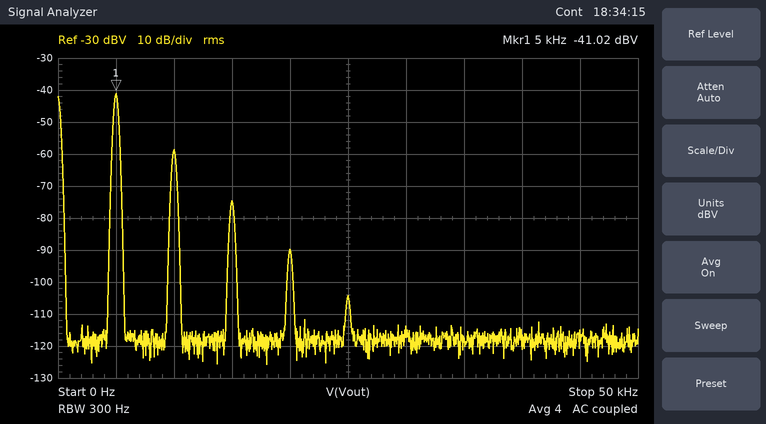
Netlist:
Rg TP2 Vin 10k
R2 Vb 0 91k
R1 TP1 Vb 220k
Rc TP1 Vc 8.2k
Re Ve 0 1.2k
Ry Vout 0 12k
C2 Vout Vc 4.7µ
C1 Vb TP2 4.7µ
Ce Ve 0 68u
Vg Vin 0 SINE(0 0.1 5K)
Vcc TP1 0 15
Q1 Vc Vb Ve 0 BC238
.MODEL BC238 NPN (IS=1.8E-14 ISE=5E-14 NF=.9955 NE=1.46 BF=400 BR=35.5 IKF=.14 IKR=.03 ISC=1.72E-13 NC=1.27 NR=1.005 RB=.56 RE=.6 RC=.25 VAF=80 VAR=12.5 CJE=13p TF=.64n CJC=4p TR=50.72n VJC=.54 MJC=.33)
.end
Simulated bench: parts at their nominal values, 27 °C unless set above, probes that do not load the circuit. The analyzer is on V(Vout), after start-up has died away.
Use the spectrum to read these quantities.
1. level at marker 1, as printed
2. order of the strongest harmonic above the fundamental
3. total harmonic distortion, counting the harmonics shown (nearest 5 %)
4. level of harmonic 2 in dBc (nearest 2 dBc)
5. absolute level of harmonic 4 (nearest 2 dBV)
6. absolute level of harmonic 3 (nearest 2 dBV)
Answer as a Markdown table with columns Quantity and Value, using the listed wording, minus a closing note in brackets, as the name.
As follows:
| Quantity | Value |
|---|---|
| level at marker 1, as printed | -41.02 dBV |
| order of the strongest harmonic above the fundamental | 2 |
| total harmonic distortion, counting the harmonics shown | 15 % |
| level of harmonic 2 in dBc | -18 dBc |
| absolute level of harmonic 4 | -90 dBV |
| absolute level of harmonic 3 | -74 dBV |
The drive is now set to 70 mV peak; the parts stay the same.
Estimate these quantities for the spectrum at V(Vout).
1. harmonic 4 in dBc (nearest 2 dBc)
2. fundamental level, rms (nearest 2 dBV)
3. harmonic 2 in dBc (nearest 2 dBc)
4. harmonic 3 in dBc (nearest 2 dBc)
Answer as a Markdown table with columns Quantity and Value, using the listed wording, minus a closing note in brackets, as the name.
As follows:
| Quantity | Value |
|---|---|
| harmonic 4 in dBc | -58 dBc |
| fundamental level, rms | -44 dBV |
| harmonic 2 in dBc | -20 dBc |
| harmonic 3 in dBc | -40 dBc |
